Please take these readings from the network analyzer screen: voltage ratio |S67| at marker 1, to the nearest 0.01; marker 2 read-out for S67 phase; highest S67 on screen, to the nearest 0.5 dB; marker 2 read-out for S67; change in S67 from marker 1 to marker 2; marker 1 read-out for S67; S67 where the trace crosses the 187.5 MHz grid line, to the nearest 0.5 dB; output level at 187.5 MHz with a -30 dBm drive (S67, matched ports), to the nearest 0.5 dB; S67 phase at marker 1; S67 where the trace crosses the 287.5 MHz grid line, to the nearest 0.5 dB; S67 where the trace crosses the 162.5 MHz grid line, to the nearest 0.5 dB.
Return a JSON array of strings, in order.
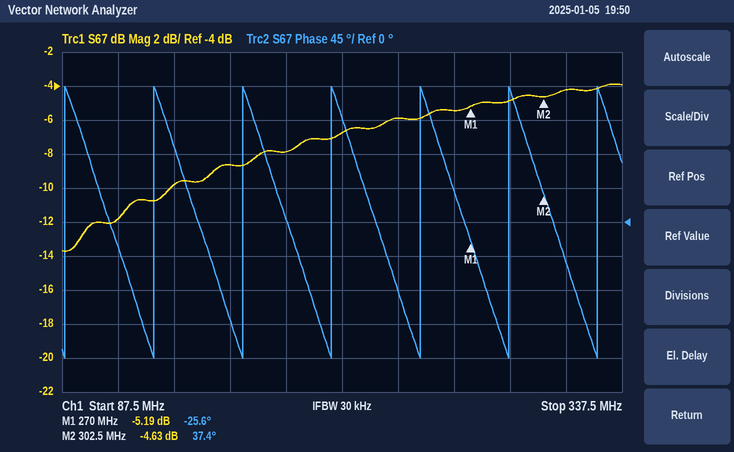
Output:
["0.55", "37.4°", "-4.0 dB", "-4.63 dB", "0.56 dB", "-5.19 dB", "-8.0 dB", "-38.0 dBm", "-25.6°", "-5.0 dB", "-8.5 dB"]
